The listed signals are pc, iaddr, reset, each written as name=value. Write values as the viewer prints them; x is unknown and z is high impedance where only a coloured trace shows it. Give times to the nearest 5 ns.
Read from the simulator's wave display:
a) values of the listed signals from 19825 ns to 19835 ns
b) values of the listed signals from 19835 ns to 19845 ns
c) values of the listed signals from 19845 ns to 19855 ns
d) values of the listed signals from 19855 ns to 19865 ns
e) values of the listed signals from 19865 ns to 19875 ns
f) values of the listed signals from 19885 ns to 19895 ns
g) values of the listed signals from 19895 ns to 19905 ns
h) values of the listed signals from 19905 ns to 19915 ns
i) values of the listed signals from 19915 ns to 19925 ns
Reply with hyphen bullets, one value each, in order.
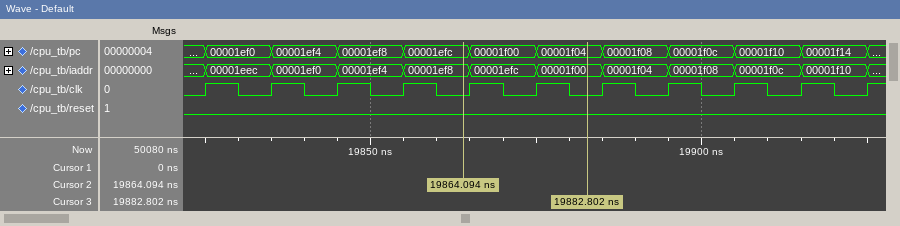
- pc=00001ef0, iaddr=00001eec, reset=0
- pc=00001ef4, iaddr=00001ef0, reset=0
- pc=00001ef8, iaddr=00001ef4, reset=0
- pc=00001efc, iaddr=00001ef8, reset=0
- pc=00001f00, iaddr=00001efc, reset=0
- pc=00001f08, iaddr=00001f04, reset=0
- pc=00001f0c, iaddr=00001f08, reset=0
- pc=00001f10, iaddr=00001f0c, reset=0
- pc=00001f14, iaddr=00001f10, reset=0
